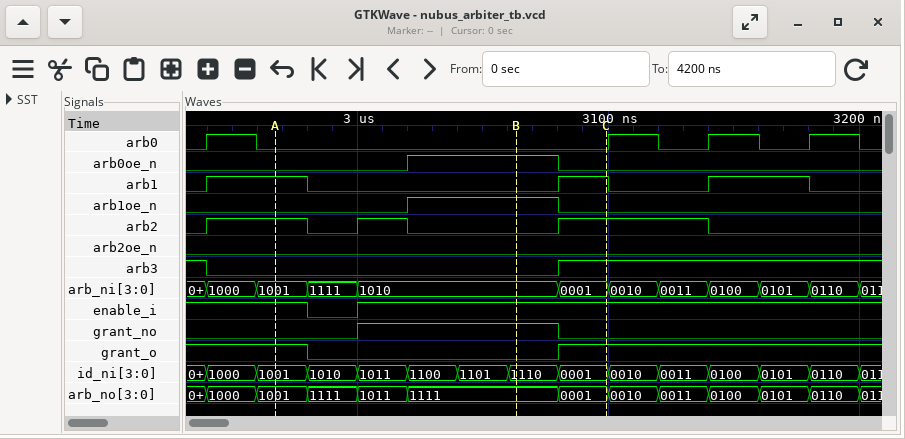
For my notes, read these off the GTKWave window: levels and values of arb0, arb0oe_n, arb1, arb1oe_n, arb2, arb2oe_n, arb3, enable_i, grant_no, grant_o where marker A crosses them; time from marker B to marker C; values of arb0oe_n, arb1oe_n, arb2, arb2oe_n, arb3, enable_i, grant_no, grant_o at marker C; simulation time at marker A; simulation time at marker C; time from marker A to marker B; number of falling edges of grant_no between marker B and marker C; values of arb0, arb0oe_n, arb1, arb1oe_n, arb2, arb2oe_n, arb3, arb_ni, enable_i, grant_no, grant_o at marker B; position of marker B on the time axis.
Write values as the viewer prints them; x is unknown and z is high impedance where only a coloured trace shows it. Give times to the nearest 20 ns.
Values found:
arb0=0, arb0oe_n=0, arb1=1, arb1oe_n=0, arb2=1, arb2oe_n=0, arb3=0, enable_i=1, grant_no=0, grant_o=1
40 ns
arb0oe_n=0, arb1oe_n=0, arb2=1, arb2oe_n=0, arb3=1, enable_i=1, grant_no=0, grant_o=1
2960 ns
3100 ns
100 ns
1
arb0=0, arb0oe_n=1, arb1=0, arb1oe_n=1, arb2=0, arb2oe_n=0, arb3=0, arb_ni=1010, enable_i=1, grant_no=1, grant_o=0
3060 ns
